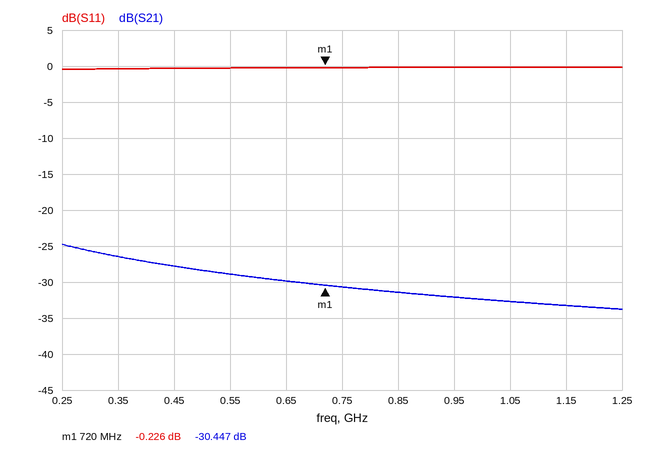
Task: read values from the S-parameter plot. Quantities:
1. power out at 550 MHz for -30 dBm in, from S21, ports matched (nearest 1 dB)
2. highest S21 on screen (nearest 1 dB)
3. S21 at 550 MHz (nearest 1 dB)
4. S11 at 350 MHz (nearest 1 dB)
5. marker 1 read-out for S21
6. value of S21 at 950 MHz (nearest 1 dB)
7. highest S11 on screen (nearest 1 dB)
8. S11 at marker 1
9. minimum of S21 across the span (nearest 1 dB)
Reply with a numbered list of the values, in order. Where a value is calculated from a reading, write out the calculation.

1. -30 dBm + (-29 dB) = -59 dBm
2. -25 dB
3. -29 dB
4. 0 dB
5. -30.447 dB
6. -32 dB
7. 0 dB
8. -0.226 dB
9. -34 dB
